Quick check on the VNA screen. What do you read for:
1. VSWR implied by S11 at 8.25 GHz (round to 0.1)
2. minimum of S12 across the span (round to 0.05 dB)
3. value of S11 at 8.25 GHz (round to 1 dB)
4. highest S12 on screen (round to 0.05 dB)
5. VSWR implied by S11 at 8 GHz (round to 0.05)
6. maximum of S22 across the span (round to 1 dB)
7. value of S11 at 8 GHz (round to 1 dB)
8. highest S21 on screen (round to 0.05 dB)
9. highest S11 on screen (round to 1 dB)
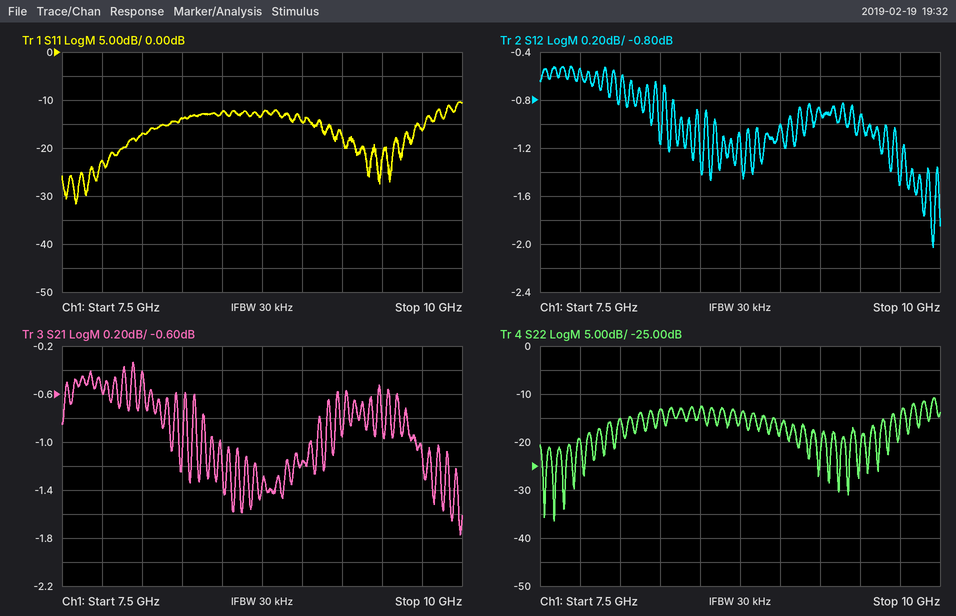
1.5
-2.05 dB
-14 dB
-0.50 dB
1.35
-11 dB
-17 dB
-0.35 dB
-10 dB
